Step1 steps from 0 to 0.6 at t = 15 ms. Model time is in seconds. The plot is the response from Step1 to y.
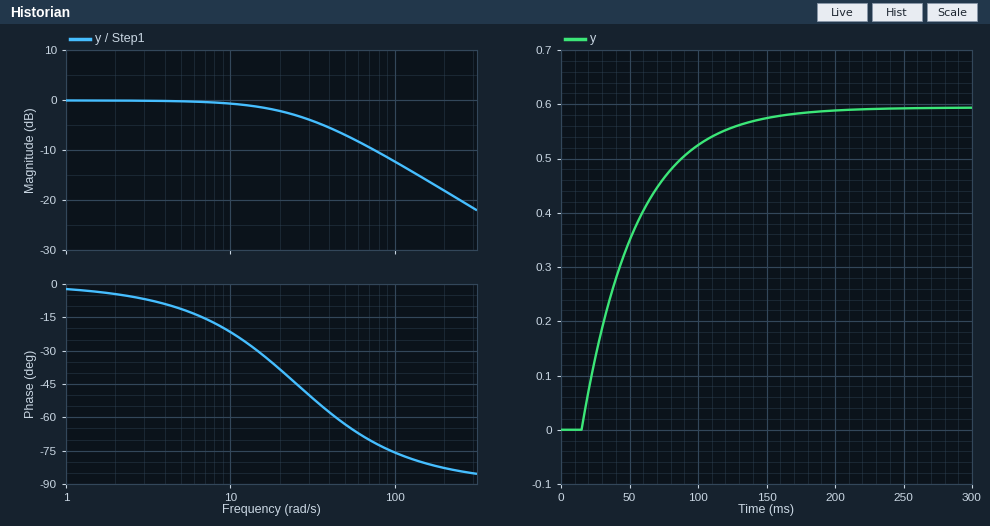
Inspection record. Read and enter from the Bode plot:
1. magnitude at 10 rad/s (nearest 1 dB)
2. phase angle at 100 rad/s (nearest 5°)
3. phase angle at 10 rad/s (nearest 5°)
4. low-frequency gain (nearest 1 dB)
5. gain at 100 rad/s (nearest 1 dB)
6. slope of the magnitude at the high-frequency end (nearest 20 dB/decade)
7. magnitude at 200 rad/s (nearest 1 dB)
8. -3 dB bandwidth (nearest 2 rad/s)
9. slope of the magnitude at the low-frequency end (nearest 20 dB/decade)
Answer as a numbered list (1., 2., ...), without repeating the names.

1. -1 dB
2. -75°
3. -20°
4. 0 dB
5. -12 dB
6. -20 dB/decade
7. -18 dB
8. 26 rad/s
9. 0 dB/decade
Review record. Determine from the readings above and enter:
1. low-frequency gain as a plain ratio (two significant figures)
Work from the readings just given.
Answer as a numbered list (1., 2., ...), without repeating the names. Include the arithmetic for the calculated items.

1. 10^(0 / 20) = 1.0
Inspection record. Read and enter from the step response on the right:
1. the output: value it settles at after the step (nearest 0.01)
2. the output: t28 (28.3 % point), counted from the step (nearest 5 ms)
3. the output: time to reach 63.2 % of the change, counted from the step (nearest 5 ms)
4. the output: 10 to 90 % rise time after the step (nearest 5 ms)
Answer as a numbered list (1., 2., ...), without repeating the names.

1. 0.59
2. 15 ms
3. 40 ms
4. 85 ms
